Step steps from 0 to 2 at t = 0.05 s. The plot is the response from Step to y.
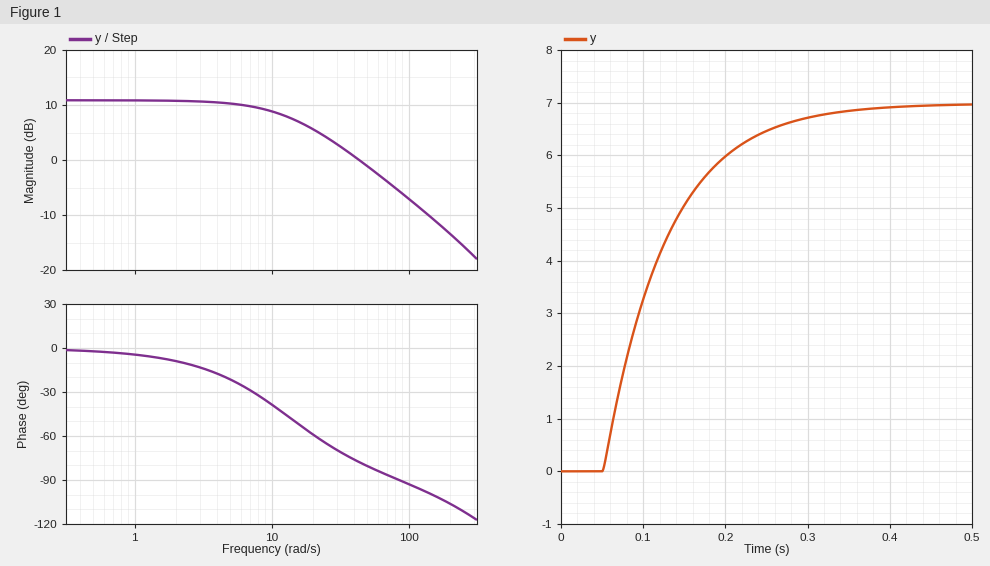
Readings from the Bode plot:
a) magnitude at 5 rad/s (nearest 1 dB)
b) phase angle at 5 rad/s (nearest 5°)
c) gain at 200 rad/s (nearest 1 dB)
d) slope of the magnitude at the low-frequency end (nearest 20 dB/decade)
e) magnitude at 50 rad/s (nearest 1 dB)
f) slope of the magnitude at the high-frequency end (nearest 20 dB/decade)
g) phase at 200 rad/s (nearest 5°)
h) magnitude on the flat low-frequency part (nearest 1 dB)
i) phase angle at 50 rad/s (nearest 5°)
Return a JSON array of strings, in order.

["10 dB", "-20°", "-13 dB", "0 dB/decade", "-1 dB", "-20 dB/decade", "-105°", "11 dB", "-80°"]
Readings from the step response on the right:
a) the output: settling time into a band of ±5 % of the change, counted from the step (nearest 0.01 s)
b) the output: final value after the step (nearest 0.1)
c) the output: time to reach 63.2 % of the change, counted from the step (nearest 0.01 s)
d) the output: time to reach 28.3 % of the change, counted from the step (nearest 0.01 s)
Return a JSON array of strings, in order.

["0.23 s", "7.0", "0.08 s", "0.03 s"]
